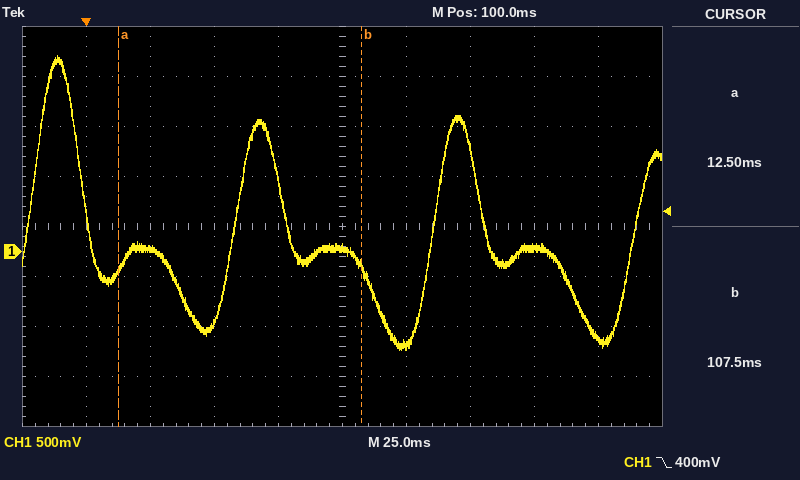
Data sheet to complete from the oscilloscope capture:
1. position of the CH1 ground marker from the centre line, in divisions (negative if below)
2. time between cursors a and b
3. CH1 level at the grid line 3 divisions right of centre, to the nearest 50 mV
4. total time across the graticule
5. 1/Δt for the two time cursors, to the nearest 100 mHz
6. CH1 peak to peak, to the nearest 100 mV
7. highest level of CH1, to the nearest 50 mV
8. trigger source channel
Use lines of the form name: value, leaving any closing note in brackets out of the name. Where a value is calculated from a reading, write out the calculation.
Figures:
position of the CH1 ground marker from the centre line, in divisions: -0.5 div
time between cursors a and b: 107.5 ms − (12.5 ms) = 95.0 ms
CH1 level at the grid line 3 divisions right of centre, to the nearest 50 mV: 50 mV
total time across the graticule: 250 ms
1/Δt for the two time cursors, to the nearest 100 mHz: 1 / 95.0 ms ≈ 10.5 Hz
CH1 peak to peak, to the nearest 100 mV: 2.90 V
highest level of CH1, to the nearest 50 mV: 1.95 V
trigger source channel: CH1
